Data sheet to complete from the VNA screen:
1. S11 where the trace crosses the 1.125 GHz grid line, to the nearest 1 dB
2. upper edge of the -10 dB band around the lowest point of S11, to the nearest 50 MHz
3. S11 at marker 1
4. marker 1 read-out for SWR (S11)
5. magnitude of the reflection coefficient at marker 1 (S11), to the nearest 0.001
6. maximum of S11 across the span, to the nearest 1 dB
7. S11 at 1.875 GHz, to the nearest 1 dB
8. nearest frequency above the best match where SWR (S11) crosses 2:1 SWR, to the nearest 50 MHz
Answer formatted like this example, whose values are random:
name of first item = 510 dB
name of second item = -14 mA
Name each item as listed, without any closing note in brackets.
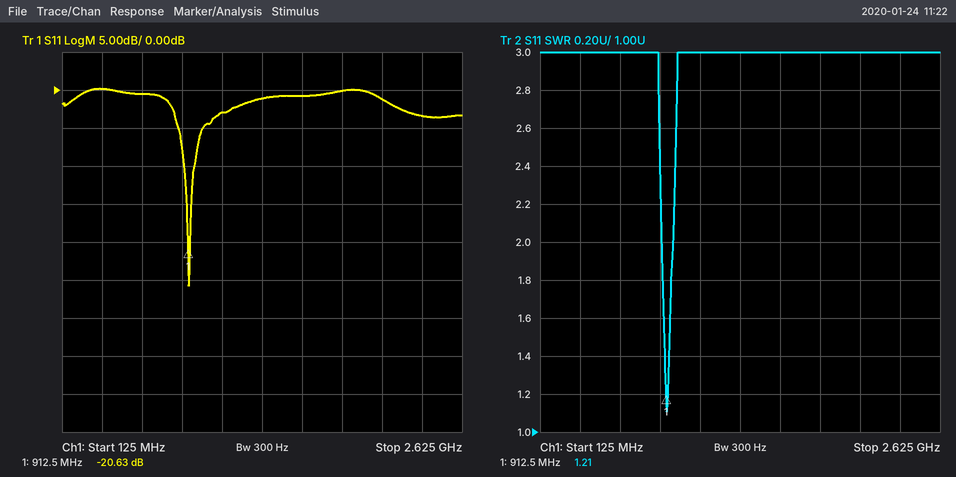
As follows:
S11 where the trace crosses the 1.125 GHz grid line, to the nearest 1 dB = -3 dB
upper edge of the -10 dB band around the lowest point of S11, to the nearest 50 MHz = 950 MHz
S11 at marker 1 = -20.63 dB
marker 1 read-out for SWR = 1.21
magnitude of the reflection coefficient at marker 1 (S11), to the nearest 0.001 = 0.093
maximum of S11 across the span, to the nearest 1 dB = 0 dB
S11 at 1.875 GHz, to the nearest 1 dB = 0 dB
nearest frequency above the best match where SWR (S11) crosses 2:1 SWR, to the nearest 50 MHz = 950 MHz
